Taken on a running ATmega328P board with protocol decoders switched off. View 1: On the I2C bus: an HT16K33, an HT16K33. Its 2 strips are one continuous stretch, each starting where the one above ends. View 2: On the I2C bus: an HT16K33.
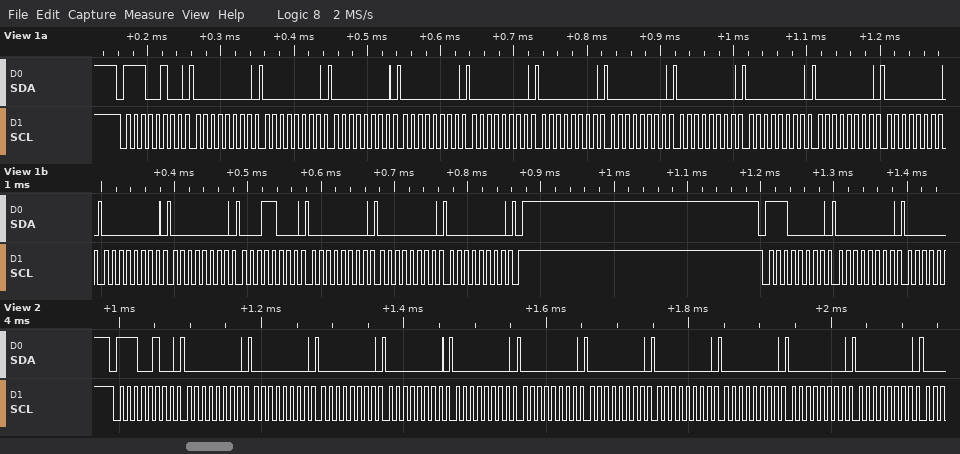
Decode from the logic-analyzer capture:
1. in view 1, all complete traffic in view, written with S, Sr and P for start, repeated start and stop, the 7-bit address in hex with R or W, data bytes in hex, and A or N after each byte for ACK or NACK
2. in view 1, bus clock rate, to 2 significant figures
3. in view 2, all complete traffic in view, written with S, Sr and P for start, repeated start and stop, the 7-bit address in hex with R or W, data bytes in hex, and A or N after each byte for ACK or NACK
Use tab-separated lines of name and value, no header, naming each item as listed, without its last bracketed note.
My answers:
in view 1, all complete traffic in view, written with S, Sr and P for start, repeated start and stop, the 7-bit address in hex with R or W, data bytes in hex, and A or N after each byte for ACK or NACK	S 72W A 00 A 00 A 00 A 00 A 00 A 00 A 00 A 00 A 00 A 00 A 00 A 00 A 00 A 18 A 00 A 00 A 00 A P S 70W A 00 A
in view 1, bus clock rate, to 2 significant figures	100 kHz
in view 2, all complete traffic in view, written with S, Sr and P for start, repeated start and stop, the 7-bit address in hex with R or W, data bytes in hex, and A or N after each byte for ACK or NACK	S 72W A 00 A 00 A 00 A 00 A 00 A 00 A 00 A 00 A 00 A 00 A 00 A
